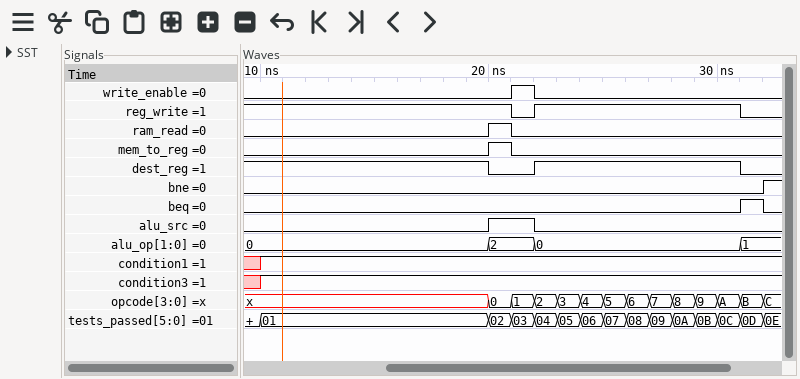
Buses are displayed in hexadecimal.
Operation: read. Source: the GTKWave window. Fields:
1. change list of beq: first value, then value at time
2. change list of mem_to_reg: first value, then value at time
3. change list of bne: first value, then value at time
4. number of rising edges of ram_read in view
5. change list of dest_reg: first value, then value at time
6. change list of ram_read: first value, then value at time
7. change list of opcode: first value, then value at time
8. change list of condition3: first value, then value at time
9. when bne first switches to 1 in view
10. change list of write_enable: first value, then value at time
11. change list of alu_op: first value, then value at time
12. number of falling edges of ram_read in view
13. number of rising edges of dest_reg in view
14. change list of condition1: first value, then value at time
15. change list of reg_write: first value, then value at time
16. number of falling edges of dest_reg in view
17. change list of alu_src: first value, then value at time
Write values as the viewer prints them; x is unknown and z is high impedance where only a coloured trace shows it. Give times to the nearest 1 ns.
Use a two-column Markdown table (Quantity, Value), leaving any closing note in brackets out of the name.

| Quantity | Value |
|---|---|
| change list of beq: first value, then value at time | 0, 1 at 31 ns, 0 at 32 ns |
| change list of mem_to_reg: first value, then value at time | 0, 1 at 20 ns, 0 at 21 ns |
| change list of bne: first value, then value at time | 0, 1 at 32 ns |
| number of rising edges of ram_read in view | 1 |
| change list of dest_reg: first value, then value at time | 1, 0 at 20 ns, 1 at 22 ns, 0 at 31 ns |
| change list of ram_read: first value, then value at time | 0, 1 at 20 ns, 0 at 21 ns |
| change list of opcode: first value, then value at time | x, 0 at 20 ns, 1 at 21 ns, 2 at 22 ns, 3 at 23 ns, 4 at 24 ns, 5 at 25 ns, 6 at 26 ns, 7 at 27 ns, 8 at 28 ns, 9 at 29 ns, A at 30 ns, B at 31 ns, C at 32 ns |
| change list of condition3: first value, then value at time | x, 1 at 10 ns |
| when bne first switches to 1 in view | 32 ns |
| change list of write_enable: first value, then value at time | 0, 1 at 21 ns, 0 at 22 ns |
| change list of alu_op: first value, then value at time | 0, 2 at 20 ns, 0 at 22 ns, 1 at 31 ns |
| number of falling edges of ram_read in view | 1 |
| number of rising edges of dest_reg in view | 1 |
| change list of condition1: first value, then value at time | x, 1 at 10 ns |
| change list of reg_write: first value, then value at time | 1, 0 at 21 ns, 1 at 22 ns, 0 at 31 ns |
| number of falling edges of dest_reg in view | 2 |
| change list of alu_src: first value, then value at time | 0, 1 at 20 ns, 0 at 22 ns |
